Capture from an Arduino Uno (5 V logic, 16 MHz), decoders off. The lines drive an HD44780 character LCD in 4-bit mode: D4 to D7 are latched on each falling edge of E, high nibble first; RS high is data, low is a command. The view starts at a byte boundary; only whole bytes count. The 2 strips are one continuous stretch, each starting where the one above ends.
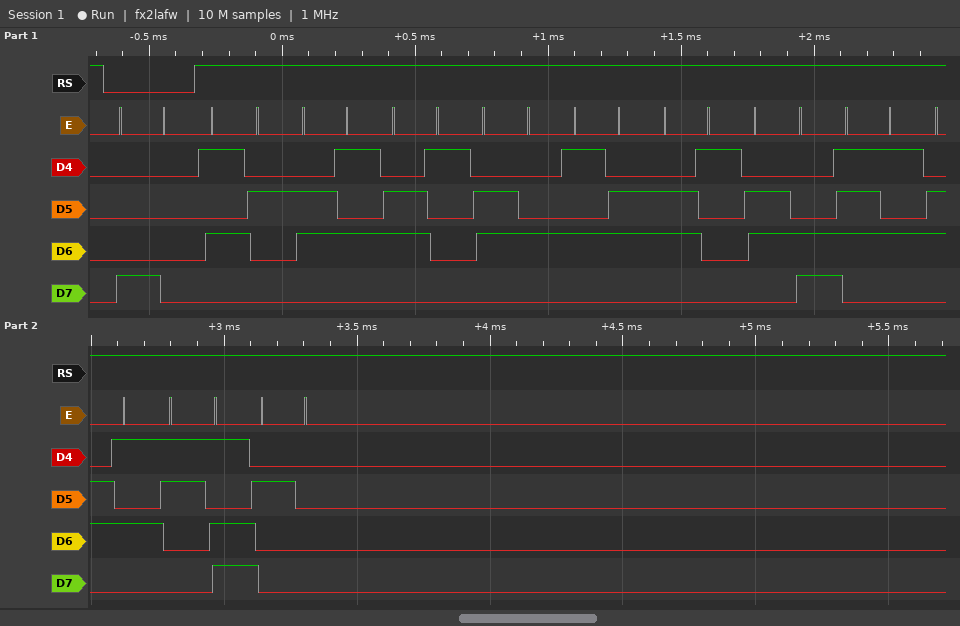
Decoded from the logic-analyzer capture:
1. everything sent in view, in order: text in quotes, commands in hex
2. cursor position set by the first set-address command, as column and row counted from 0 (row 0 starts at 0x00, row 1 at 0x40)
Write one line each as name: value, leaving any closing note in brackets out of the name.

everything sent in view, in order: text in quotes, commands in hex: 0x80 "ReadValue= "
cursor position set by the first set-address command, as column and row counted from 0: column 0, row 0
